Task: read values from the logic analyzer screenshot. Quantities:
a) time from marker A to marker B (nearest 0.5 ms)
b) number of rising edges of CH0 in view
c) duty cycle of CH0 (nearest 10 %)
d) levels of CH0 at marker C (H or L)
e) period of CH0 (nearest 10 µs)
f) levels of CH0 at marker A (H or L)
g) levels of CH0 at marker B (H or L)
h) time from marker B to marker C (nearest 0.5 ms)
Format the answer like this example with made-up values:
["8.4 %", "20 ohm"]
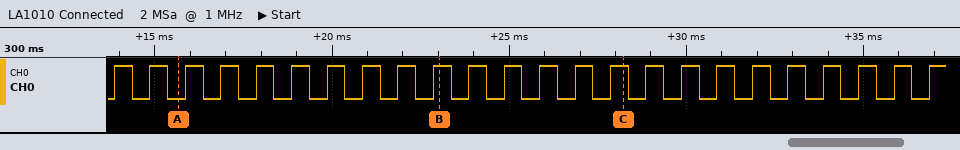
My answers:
["7.5 ms", "24", "50 %", "CH0=H", "1000 µs", "CH0=L", "CH0=H", "5 ms"]
